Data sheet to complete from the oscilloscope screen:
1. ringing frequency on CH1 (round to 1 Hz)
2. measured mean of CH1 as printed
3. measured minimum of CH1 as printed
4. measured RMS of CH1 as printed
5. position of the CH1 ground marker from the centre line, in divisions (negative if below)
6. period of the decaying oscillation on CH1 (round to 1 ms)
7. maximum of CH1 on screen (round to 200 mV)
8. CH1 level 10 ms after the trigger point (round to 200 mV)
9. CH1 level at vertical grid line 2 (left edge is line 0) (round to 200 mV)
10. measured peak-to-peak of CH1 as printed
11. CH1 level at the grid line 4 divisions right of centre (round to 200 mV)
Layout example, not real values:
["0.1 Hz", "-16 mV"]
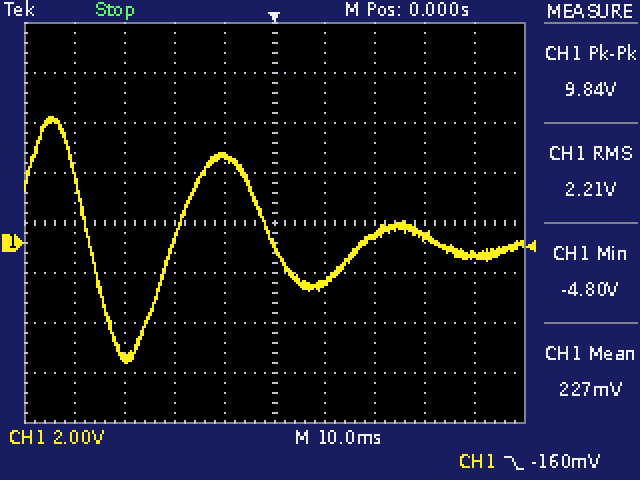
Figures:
["29 Hz", "227 mV", "-4.80 V", "2.21 V", "-0.4 div", "35 ms", "5.0 V", "-1.6 V", "-4.6 V", "9.84 V", "-400 mV"]
